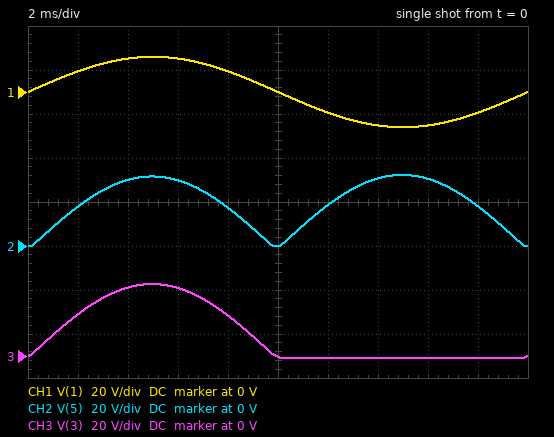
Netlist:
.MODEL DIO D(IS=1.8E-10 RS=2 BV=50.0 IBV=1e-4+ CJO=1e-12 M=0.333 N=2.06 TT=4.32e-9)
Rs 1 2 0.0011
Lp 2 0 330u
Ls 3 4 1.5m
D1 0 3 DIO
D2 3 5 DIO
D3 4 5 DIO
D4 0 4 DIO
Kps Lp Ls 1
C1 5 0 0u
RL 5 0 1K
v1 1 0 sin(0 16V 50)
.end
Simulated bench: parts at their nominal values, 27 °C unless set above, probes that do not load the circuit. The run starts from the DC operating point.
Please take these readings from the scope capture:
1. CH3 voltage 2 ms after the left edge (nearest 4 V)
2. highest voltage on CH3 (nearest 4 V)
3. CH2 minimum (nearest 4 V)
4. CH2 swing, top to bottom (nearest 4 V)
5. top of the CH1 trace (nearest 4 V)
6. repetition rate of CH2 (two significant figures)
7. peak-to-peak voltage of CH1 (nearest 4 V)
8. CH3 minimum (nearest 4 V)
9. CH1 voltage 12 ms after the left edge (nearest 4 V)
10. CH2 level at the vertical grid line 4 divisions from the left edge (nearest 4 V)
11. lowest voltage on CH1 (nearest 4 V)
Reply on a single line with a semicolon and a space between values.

20 V; 32 V; 0 V; 32 V; 16 V; 100 Hz; 32 V; 0 V; -8 V; 16 V; -16 V
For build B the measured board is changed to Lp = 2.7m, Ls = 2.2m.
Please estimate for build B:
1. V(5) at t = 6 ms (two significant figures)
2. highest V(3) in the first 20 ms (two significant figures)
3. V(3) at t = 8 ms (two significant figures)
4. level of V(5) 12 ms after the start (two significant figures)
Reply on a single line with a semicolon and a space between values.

12 V; 13 V; 7.5 V; 6.6 V
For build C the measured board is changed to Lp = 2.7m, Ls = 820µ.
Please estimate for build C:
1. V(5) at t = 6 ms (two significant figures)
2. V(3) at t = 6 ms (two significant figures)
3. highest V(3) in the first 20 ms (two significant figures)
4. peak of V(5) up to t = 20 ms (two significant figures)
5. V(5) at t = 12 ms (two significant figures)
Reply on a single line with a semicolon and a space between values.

6.5 V; 7.4 V; 7.9 V; 6.9 V; 3.4 V
